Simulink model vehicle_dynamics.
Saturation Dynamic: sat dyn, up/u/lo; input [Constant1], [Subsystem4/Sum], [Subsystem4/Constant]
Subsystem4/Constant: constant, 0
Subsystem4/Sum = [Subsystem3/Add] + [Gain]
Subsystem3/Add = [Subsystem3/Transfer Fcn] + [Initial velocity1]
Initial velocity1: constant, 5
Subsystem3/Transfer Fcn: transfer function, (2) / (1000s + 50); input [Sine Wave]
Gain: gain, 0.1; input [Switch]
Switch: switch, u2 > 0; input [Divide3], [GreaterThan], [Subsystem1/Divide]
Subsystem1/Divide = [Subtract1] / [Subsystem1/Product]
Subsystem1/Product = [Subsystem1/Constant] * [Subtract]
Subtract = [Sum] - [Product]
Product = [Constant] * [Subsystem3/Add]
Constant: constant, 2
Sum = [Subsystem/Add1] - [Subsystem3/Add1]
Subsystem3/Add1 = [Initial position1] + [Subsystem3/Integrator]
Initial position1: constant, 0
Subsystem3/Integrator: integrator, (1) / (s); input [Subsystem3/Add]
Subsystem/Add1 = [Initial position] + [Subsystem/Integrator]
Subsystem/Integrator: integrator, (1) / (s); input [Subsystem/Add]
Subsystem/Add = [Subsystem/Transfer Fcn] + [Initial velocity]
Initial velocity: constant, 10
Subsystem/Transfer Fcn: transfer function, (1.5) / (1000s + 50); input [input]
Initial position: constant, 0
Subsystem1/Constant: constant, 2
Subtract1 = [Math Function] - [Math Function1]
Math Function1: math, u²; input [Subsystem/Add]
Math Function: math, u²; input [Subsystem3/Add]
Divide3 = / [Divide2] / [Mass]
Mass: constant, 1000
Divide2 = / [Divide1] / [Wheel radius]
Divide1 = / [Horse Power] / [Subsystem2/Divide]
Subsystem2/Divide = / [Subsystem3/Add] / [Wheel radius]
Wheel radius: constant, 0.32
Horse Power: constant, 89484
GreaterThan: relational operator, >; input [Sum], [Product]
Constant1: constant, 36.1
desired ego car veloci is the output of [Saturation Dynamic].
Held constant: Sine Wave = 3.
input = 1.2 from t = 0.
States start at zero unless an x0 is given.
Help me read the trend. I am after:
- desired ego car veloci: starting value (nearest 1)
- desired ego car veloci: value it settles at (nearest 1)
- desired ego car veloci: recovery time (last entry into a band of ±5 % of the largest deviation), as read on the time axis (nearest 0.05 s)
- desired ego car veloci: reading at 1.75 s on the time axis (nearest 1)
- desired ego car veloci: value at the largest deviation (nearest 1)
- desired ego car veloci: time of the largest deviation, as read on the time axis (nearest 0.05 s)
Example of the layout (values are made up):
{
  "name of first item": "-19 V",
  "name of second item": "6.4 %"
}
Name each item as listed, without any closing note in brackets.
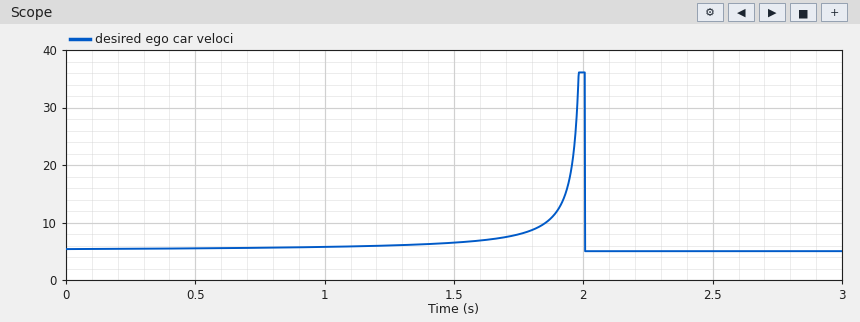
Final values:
{
  "desired ego car veloci: starting value": "5",
  "desired ego car veloci: value it settles at": "5",
  "desired ego car veloci: recovery time (last entry into a band of ±5 % of the largest deviation), as read on the time axis": "2.00 s",
  "desired ego car veloci: reading at 1.75 s on the time axis": "8",
  "desired ego car veloci: value at the largest deviation": "36",
  "desired ego car veloci: time of the largest deviation, as read on the time axis": "2.00 s"
}
